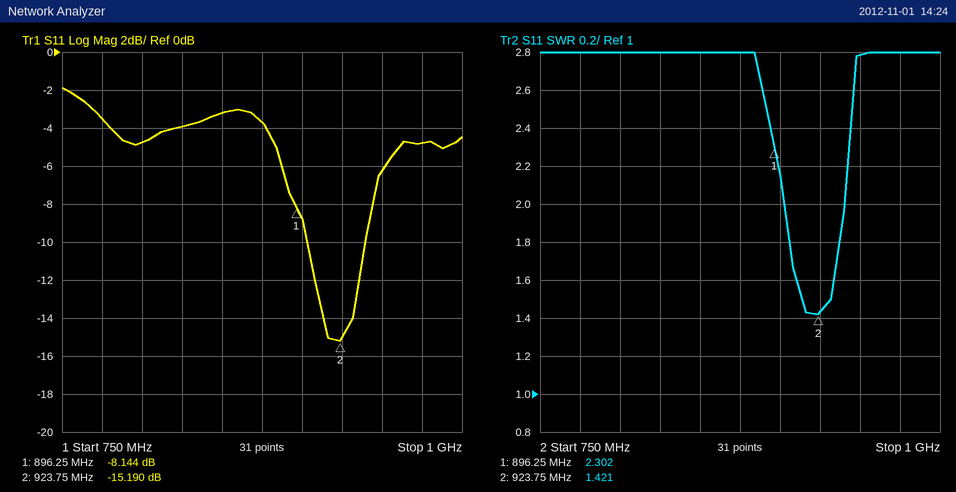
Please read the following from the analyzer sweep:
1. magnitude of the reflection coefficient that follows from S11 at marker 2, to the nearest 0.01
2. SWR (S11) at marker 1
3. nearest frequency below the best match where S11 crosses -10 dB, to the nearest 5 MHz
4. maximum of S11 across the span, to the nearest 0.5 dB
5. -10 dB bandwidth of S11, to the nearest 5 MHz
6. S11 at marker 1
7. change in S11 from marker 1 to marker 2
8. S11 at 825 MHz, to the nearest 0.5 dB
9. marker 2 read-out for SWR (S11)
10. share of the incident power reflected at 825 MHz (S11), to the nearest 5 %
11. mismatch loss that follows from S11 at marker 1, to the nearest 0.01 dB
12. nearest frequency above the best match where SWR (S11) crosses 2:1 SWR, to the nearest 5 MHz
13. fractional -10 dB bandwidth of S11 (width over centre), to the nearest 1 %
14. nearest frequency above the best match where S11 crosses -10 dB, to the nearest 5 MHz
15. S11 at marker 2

0.17
2.302
905 MHz
-2.0 dB
35 MHz
-8.144 dB
-7.046 dB
-4.0 dB
1.421
40 %
0.72 dB
940 MHz
4 %
940 MHz
-15.190 dB
